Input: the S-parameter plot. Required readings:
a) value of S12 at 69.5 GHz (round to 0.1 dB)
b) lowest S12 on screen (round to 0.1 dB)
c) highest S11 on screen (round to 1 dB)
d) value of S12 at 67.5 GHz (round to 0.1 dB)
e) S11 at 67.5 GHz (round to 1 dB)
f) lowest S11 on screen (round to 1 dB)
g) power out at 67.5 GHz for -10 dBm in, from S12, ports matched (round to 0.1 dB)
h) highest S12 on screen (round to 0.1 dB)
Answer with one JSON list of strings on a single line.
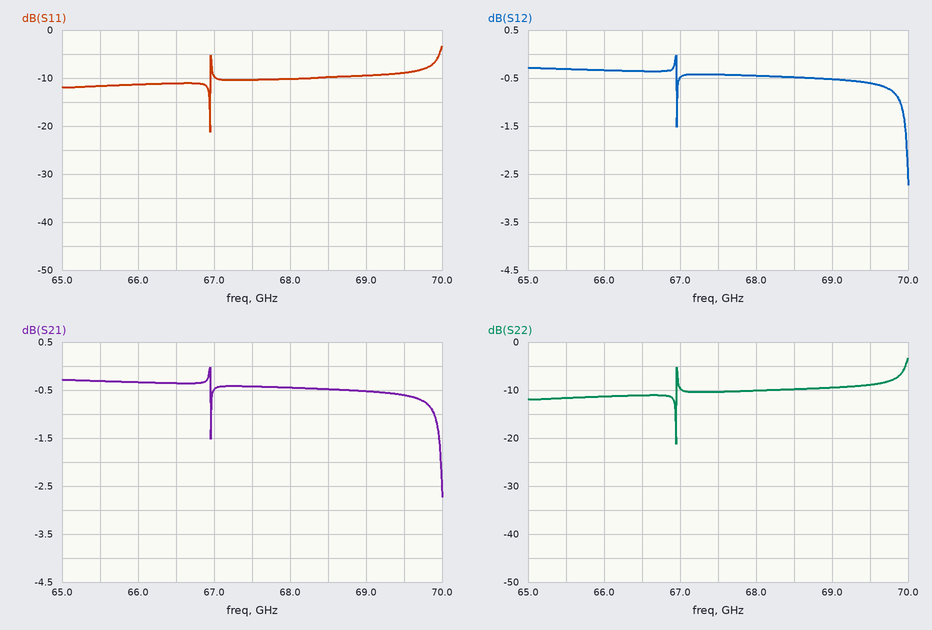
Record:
["-0.6 dB", "-2.7 dB", "-3 dB", "-0.4 dB", "-10 dB", "-21 dB", "-10.4 dBm", "0.0 dB"]
